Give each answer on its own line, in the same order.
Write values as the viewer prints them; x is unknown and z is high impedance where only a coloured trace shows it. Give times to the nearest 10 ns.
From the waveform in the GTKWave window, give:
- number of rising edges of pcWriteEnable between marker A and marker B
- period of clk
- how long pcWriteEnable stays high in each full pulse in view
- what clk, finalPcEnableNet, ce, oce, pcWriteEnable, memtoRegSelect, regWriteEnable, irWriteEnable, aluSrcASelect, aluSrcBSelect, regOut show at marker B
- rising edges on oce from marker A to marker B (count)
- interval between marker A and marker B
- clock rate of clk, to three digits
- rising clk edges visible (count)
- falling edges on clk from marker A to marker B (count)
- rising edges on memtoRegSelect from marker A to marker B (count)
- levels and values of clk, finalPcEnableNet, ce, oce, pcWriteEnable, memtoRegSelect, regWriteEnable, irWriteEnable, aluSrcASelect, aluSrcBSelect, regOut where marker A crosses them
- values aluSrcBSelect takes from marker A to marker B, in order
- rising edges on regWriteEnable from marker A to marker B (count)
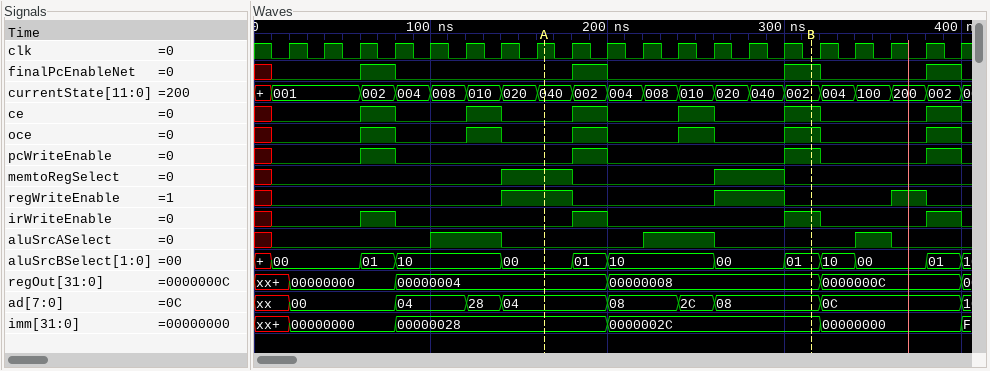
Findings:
2
20 ns
20 ns, 20 ns, 20 ns, 20 ns
clk=0, finalPcEnableNet=1, ce=1, oce=1, pcWriteEnable=1, memtoRegSelect=0, regWriteEnable=0, irWriteEnable=1, aluSrcASelect=0, aluSrcBSelect=01, regOut=00000008
3
150 ns
50.0 MHz
20
8
1
clk=1, finalPcEnableNet=0, ce=0, oce=0, pcWriteEnable=0, memtoRegSelect=1, regWriteEnable=1, irWriteEnable=0, aluSrcASelect=0, aluSrcBSelect=00, regOut=00000004
00, 01, 10, 00, 01
1
